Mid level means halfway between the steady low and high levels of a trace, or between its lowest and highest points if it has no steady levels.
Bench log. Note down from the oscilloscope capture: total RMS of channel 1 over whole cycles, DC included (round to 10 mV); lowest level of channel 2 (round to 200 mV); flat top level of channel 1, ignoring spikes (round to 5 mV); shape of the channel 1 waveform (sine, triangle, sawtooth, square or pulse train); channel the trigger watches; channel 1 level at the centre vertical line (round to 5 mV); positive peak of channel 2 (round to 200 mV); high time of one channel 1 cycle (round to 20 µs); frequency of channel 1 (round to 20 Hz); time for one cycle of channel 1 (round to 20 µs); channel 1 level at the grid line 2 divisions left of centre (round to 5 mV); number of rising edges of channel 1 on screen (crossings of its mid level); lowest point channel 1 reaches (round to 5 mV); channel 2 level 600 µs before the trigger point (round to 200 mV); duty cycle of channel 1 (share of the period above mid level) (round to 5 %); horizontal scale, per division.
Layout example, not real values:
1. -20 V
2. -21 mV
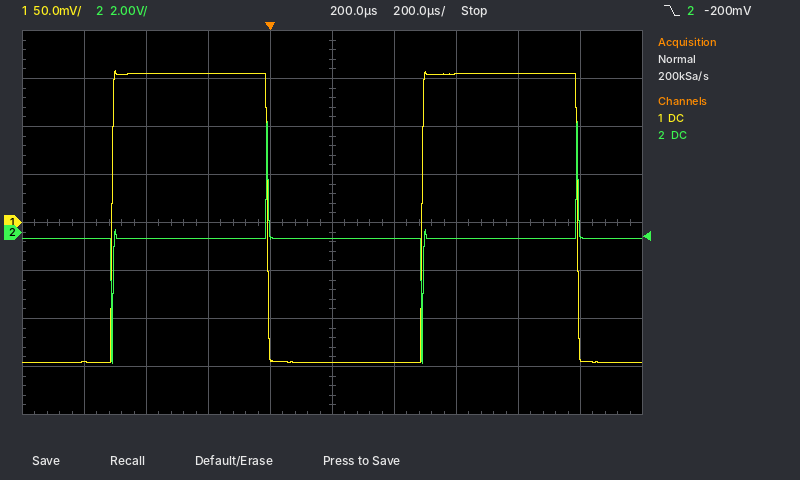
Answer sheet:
1. 150 mV
2. -5.4 V
3. 155 mV
4. square
5. channel 2
6. -145 mV
7. 4.6 V
8. 500 µs
9. 1.00 kHz
10. 1.00 ms
11. 155 mV
12. 2
13. -145 mV
14. -200 mV
15. 50 %
16. 200 µs
